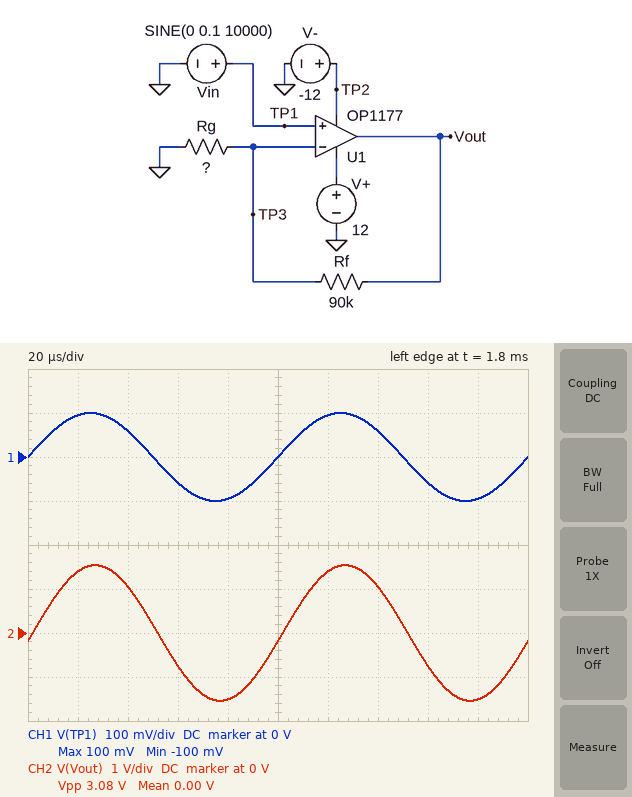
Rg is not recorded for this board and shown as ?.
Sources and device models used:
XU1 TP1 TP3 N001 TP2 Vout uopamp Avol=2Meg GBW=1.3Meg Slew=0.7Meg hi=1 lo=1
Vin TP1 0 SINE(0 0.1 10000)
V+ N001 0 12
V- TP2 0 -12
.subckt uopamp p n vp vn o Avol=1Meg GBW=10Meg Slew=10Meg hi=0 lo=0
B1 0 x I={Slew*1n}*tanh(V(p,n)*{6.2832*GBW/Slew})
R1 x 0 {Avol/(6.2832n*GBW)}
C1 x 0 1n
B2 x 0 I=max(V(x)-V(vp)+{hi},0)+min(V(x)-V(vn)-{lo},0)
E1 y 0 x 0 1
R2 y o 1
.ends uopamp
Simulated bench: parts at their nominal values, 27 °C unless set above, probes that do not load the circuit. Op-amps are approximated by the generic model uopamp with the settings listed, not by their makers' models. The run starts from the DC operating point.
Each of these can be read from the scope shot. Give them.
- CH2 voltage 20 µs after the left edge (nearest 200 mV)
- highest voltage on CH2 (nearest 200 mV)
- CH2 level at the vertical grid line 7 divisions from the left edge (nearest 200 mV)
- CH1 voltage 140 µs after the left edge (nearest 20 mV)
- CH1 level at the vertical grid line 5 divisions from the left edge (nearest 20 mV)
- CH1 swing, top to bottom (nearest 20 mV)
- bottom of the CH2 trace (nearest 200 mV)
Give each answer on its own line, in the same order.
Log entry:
1.4 V
1.6 V
1.0 V
60 mV
0 V
200 mV
-1.6 V
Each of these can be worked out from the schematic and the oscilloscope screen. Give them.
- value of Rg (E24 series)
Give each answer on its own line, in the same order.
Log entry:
6.2 kΩ
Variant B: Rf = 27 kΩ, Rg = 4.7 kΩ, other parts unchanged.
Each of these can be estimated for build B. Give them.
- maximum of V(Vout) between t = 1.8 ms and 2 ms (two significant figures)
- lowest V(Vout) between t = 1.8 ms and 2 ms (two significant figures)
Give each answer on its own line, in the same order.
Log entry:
670 mV
-670 mV
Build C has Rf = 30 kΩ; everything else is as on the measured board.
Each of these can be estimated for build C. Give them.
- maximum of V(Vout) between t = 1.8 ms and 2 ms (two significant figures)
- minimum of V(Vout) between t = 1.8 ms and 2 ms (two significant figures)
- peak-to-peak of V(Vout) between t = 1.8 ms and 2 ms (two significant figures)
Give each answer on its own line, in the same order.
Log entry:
580 mV
-580 mV
1.2 V
